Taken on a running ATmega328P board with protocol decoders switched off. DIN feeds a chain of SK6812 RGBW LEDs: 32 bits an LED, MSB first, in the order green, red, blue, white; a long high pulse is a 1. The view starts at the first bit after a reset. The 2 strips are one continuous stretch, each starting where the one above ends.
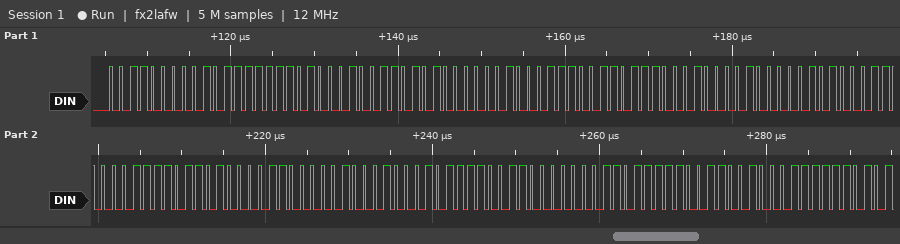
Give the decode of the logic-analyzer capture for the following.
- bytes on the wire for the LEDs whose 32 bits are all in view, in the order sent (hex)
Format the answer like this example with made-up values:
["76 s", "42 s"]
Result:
["30 5F D1 35 02 39 B8 84 14 61 ED 0C 11 17 98 0D"]
